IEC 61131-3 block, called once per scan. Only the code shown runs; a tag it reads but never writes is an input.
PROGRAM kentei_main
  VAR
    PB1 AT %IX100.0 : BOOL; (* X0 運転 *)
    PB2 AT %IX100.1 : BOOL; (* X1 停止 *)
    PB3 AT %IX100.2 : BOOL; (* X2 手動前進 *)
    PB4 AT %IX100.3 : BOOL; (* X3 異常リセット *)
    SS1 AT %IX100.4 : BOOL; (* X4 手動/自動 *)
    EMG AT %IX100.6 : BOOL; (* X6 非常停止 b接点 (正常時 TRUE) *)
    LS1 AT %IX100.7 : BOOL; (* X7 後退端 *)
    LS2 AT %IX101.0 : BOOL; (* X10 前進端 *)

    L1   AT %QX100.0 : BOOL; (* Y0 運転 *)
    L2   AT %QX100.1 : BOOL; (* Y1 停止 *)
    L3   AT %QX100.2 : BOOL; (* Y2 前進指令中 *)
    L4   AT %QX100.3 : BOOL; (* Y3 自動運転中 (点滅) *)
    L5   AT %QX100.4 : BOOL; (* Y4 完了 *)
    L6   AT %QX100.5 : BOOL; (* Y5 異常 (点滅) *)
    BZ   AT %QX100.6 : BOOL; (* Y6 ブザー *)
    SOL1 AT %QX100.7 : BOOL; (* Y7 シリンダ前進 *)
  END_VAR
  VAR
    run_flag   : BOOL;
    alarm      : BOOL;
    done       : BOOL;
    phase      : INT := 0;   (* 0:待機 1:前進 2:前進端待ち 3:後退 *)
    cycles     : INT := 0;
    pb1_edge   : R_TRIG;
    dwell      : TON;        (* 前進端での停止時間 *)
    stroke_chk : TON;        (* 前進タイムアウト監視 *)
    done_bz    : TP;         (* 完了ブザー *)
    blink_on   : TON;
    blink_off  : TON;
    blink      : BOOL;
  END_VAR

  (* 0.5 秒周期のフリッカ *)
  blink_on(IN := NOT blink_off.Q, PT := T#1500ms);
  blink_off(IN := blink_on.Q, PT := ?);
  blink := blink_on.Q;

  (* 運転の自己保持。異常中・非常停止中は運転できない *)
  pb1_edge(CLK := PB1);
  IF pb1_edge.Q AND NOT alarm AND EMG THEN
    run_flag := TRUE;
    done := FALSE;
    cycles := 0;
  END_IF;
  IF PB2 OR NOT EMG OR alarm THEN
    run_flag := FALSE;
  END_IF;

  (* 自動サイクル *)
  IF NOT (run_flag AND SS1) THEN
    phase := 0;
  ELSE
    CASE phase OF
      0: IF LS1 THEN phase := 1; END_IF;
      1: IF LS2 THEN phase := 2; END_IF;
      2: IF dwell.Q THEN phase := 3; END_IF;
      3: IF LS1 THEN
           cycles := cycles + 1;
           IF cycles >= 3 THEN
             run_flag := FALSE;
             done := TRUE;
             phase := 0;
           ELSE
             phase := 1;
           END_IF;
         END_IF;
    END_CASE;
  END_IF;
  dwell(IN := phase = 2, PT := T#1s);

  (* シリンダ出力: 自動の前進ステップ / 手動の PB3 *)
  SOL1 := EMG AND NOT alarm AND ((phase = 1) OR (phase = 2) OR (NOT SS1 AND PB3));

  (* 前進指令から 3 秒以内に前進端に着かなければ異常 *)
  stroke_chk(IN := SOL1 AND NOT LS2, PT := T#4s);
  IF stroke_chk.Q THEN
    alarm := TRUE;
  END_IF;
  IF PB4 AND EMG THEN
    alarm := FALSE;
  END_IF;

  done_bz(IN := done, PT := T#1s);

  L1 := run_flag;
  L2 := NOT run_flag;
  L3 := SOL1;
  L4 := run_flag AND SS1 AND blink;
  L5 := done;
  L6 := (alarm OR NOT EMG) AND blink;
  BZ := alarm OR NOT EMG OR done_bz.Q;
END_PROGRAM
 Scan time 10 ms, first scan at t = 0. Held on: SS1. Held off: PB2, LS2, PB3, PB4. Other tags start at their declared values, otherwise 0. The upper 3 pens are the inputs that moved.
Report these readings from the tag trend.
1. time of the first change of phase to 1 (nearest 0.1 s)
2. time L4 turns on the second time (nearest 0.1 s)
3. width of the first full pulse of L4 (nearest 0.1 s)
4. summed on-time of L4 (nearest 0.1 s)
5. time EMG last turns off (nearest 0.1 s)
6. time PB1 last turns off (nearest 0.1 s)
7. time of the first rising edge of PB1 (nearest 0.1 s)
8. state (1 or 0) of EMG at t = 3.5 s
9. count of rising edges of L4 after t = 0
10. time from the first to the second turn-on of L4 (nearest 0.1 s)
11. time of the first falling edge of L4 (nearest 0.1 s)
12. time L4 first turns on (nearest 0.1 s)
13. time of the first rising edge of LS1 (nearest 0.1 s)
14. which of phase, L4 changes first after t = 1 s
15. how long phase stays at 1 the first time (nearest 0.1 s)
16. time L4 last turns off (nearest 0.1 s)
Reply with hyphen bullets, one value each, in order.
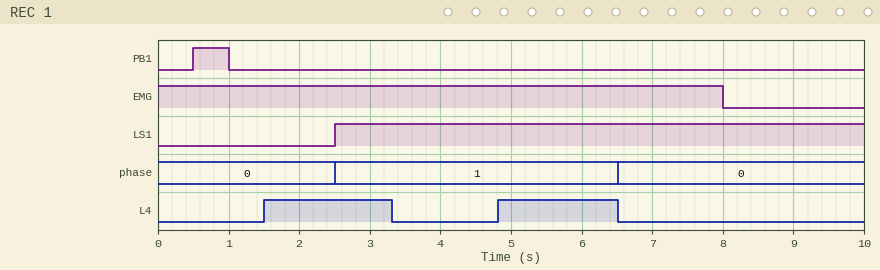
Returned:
- 2.5 s
- 4.8 s
- 1.8 s
- 3.5 s
- 8.0 s
- 1.0 s
- 0.5 s
- 1
- 2
- 3.3 s
- 3.3 s
- 1.5 s
- 2.5 s
- L4
- 4.0 s
- 6.5 s
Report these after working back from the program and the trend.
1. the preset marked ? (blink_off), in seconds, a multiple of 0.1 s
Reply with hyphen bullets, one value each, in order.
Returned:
- 1.8 s
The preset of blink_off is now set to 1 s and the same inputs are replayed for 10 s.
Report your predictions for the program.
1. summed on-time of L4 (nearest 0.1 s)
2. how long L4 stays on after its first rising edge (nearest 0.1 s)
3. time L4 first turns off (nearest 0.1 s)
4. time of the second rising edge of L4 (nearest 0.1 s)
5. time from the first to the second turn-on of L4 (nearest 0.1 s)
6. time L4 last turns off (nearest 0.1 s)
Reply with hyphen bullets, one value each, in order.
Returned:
- 2.0 s
- 1.0 s
- 2.5 s
- 4.0 s
- 2.5 s
- 5.0 s
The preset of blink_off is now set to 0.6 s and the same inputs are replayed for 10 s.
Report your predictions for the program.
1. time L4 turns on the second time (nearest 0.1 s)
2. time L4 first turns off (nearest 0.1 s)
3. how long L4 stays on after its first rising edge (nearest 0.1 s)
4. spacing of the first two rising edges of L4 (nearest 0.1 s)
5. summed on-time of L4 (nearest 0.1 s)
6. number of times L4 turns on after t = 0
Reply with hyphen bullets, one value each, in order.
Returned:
- 3.6 s
- 2.1 s
- 0.6 s
- 2.1 s
- 1.8 s
- 3
